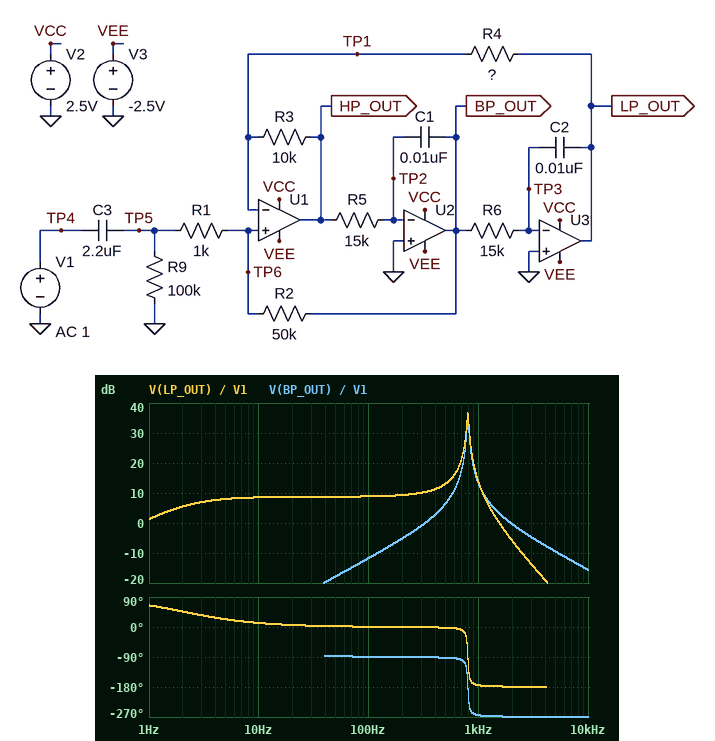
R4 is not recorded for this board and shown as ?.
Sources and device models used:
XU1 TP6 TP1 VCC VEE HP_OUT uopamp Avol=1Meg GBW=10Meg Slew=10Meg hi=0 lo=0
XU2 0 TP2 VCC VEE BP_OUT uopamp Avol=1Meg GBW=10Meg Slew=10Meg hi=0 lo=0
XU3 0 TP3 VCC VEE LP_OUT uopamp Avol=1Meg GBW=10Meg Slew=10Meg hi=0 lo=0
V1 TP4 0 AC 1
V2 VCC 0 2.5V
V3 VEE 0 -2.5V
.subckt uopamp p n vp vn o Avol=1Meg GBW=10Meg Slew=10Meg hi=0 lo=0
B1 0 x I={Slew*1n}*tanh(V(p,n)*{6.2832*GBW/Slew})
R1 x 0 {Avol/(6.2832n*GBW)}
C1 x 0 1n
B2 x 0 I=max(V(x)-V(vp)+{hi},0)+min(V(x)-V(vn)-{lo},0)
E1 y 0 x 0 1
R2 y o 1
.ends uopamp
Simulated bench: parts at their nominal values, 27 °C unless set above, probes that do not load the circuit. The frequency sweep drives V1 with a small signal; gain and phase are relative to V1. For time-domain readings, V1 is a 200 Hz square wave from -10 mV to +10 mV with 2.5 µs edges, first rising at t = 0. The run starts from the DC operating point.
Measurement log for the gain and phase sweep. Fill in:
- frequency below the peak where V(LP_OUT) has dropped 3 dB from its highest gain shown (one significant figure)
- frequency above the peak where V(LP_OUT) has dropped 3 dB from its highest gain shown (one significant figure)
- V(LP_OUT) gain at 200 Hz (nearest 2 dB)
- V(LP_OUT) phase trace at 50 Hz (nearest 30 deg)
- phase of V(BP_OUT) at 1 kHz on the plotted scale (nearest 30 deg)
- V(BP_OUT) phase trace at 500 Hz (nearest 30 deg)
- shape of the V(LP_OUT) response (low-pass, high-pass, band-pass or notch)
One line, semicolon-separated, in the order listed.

800 Hz; 800 Hz; 10 dB; 0 deg; -270 deg; -90 deg; band-pass
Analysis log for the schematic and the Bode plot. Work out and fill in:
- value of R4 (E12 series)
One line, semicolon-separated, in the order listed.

18 kΩ
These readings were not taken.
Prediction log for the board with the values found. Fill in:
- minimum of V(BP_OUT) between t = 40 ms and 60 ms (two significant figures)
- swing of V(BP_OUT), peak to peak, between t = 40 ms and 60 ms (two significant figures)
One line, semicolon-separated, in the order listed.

-22 mV; 45 mV
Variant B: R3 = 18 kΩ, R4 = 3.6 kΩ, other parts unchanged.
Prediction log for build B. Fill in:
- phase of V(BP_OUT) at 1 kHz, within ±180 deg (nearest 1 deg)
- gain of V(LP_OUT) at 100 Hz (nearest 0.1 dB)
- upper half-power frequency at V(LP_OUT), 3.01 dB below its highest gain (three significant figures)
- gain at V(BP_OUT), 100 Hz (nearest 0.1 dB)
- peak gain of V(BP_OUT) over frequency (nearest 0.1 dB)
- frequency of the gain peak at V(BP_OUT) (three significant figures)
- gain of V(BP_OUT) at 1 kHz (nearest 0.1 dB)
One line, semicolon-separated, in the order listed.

-91 deg; 1.4 dB; 2.43 kHz; -19.1 dB; 34.3 dB; 2.37 kHz; 2.6 dB
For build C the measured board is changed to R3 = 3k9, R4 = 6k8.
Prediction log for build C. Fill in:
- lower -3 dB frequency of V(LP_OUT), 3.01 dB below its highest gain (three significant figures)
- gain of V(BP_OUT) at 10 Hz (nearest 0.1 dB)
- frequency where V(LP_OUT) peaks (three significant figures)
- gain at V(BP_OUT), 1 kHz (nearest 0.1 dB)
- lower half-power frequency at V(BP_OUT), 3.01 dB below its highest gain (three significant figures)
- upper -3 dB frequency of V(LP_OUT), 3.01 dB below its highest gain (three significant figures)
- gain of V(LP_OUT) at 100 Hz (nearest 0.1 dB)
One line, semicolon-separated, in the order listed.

788 Hz; -32.1 dB; 805 Hz; 13.3 dB; 789 Hz; 821 Hz; 8.7 dB
